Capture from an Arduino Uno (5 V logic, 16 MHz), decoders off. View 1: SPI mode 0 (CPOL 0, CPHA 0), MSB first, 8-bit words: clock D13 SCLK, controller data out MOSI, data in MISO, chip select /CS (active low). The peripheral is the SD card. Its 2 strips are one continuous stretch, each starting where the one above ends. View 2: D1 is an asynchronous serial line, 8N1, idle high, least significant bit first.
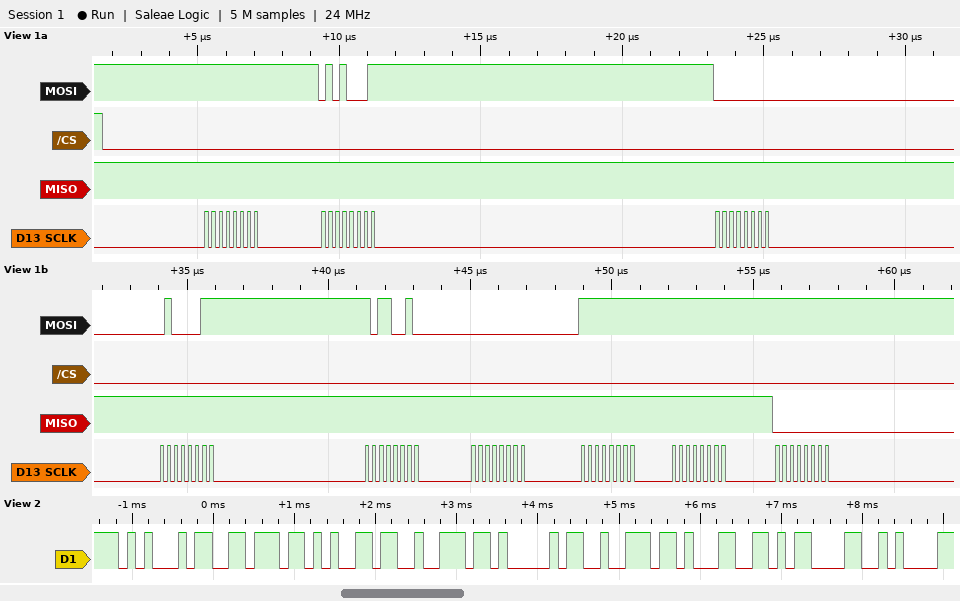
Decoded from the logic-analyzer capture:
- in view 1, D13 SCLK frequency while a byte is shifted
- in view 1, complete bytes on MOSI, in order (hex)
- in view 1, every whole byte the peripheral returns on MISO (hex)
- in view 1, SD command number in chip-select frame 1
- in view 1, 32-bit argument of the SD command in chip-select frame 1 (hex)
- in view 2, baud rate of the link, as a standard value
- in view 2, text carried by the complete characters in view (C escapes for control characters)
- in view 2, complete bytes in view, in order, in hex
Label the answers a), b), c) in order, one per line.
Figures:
a) 4 MHz
b) FF 51 00 43 B2 00 FF FF FF
c) FF FF FF FF FF FF FF FF 00
d) CMD17
e) 0x0043B200
f) 9600 baud
g) "EverAr1\r\n"
h) 45 76 65 72 41 72 31 0D 0A
